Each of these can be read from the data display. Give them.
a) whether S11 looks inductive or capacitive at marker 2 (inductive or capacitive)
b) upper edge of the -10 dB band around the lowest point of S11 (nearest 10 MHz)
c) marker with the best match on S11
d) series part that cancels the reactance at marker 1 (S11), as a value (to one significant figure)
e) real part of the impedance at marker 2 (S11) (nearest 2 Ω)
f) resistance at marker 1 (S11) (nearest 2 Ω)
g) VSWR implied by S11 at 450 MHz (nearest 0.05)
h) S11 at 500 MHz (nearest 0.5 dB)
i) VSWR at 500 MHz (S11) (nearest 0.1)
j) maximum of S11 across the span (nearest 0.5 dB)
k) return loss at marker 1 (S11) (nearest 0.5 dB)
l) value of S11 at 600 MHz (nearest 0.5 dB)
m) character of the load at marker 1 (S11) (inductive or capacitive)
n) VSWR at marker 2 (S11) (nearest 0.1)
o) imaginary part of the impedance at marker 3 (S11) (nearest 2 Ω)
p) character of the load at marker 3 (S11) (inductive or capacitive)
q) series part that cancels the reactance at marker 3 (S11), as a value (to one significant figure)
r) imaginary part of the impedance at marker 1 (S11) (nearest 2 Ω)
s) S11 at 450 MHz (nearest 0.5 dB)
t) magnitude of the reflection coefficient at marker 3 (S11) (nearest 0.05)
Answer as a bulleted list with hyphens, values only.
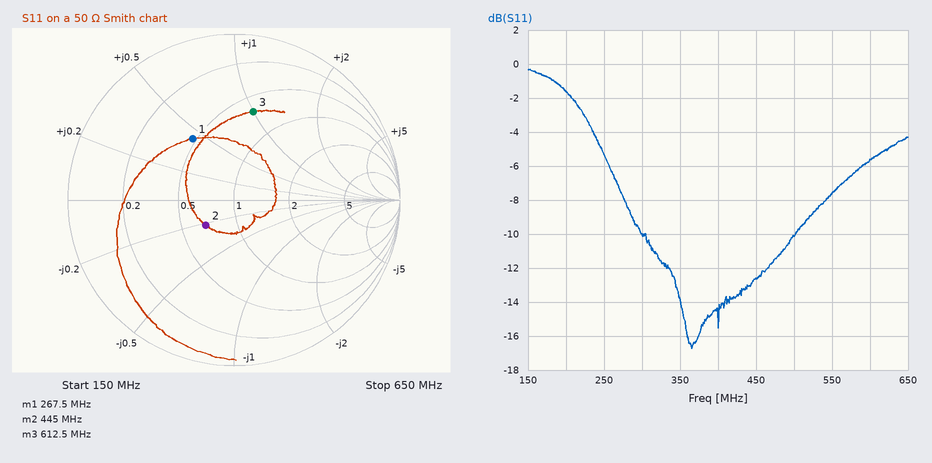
- capacitive
- 500 MHz
- marker 2
- 30 pF
- 34 Ω
- 24 Ω
- 1.60
- -10.0 dB
- 1.9
- -0.5 dB
- 7.0 dB
- -5.5 dB
- inductive
- 1.6
- +50 Ω
- inductive
- 5 pF
- +22 Ω
- -12.5 dB
- 0.55
